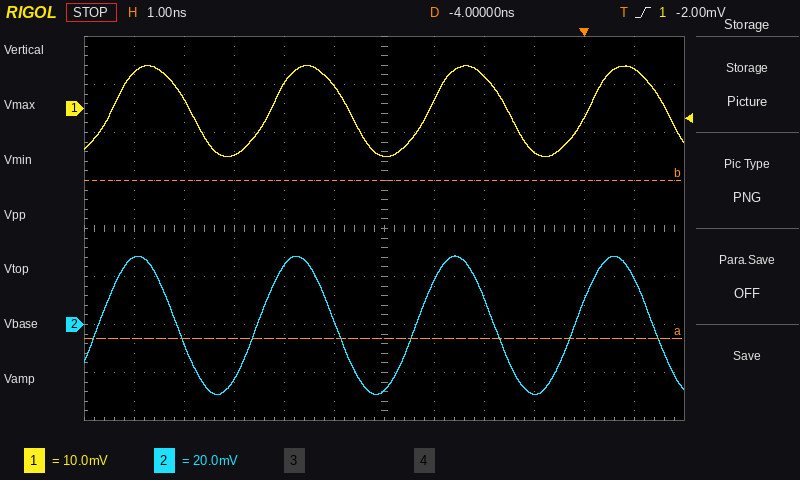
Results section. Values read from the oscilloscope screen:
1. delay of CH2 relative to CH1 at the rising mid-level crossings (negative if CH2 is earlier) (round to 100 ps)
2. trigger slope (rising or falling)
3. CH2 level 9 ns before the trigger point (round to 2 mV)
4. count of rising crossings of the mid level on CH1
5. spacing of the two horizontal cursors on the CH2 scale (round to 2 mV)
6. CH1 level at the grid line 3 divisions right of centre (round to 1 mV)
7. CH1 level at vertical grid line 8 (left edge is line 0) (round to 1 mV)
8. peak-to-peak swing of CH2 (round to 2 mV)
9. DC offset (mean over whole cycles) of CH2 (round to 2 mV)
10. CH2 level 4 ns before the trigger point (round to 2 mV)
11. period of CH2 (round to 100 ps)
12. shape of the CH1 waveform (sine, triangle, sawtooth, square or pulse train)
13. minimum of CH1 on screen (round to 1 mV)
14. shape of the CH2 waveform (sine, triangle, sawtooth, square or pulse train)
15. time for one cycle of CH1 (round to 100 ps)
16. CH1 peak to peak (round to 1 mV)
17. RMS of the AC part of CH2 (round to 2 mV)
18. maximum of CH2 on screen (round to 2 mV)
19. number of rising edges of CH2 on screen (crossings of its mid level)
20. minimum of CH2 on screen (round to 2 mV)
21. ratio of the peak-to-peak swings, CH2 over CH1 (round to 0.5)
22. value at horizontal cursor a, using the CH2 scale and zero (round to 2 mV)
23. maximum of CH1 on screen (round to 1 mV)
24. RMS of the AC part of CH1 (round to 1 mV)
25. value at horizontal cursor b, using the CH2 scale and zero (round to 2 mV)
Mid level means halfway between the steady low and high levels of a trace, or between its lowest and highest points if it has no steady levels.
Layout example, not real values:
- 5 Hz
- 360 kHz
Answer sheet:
- -300 ps
- rising
- 28 mV
- 4
- 66 mV
- -9 mV
- 7 mV
- 58 mV
- 0 mV
- -28 mV
- 3.2 ns
- sine
- -10 mV
- sine
- 3.2 ns
- 19 mV
- 20 mV
- 28 mV
- 4
- -30 mV
- 3.0
- -6 mV
- 9 mV
- 7 mV
- 60 mV
